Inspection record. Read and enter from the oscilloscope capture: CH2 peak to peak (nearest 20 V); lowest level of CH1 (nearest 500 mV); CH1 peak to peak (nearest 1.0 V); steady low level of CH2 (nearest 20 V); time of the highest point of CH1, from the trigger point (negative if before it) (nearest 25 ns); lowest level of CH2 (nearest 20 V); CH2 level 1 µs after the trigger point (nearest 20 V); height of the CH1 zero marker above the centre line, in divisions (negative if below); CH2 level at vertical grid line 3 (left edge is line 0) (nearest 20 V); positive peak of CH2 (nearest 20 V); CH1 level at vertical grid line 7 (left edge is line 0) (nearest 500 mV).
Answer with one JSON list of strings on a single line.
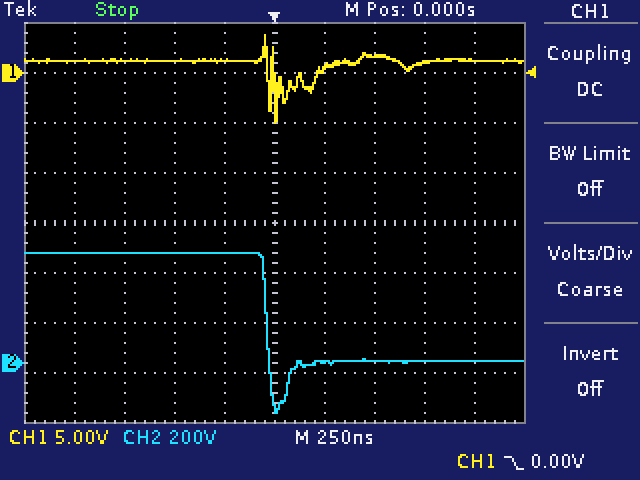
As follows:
["640 V", "-5.0 V", "9.0 V", "0 V", "-50 ns", "-200 V", "0 V", "+3.0 div", "440 V", "440 V", "1.5 V"]
